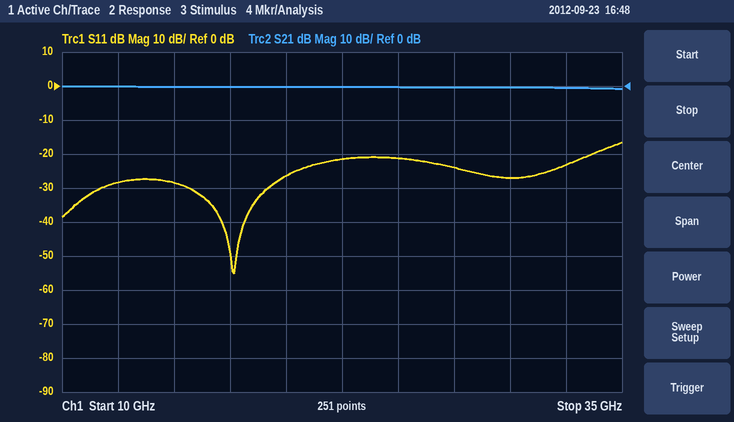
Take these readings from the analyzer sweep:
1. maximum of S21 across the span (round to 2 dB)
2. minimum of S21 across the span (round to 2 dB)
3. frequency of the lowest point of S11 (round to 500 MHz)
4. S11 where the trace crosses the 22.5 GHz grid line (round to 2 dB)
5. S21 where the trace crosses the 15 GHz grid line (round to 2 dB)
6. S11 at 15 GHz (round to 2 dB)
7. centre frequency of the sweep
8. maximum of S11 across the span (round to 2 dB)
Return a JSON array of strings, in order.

["0 dB", "0 dB", "17.5 GHz", "-22 dB", "0 dB", "-28 dB", "22.5 GHz", "-16 dB"]
